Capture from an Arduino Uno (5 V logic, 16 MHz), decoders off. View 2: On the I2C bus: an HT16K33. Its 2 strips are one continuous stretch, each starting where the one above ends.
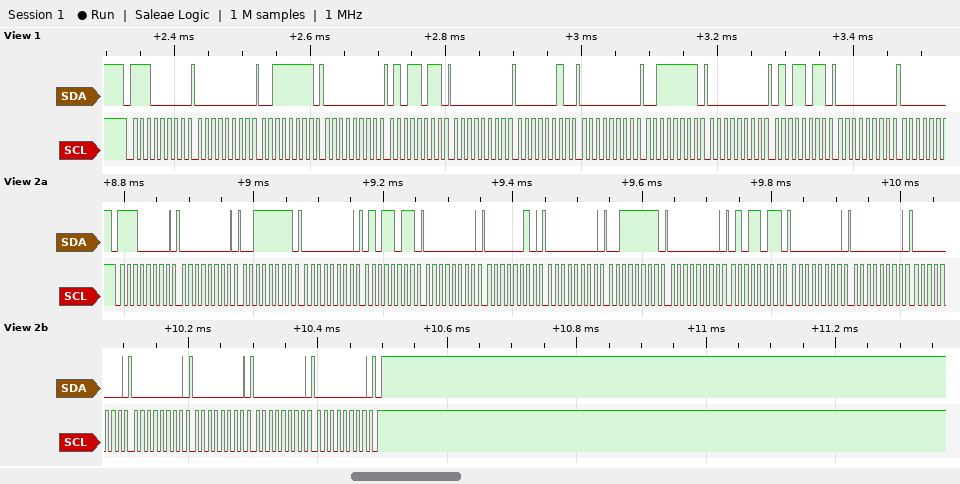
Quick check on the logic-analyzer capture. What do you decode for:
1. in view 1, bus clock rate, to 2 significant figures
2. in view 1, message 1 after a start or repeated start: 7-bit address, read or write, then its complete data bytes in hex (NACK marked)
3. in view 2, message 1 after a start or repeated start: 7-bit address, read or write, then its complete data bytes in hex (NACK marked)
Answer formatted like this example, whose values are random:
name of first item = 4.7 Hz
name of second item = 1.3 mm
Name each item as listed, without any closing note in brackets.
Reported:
in view 1, bus clock rate, to 2 significant figures = 100 kHz
in view 1, message 1 after a start or repeated start: 7-bit address, read or write, then its complete data bytes in hex = 0x70 write: 00 3F 00 5B 00 02 00 3F 00 5B 00
in view 2, message 1 after a start or repeated start: 7-bit address, read or write, then its complete data bytes in hex = 0x70 write: 00 3F 00 5B 00 02 00 3F 00 5B 00 00 00 00 00 00 00
